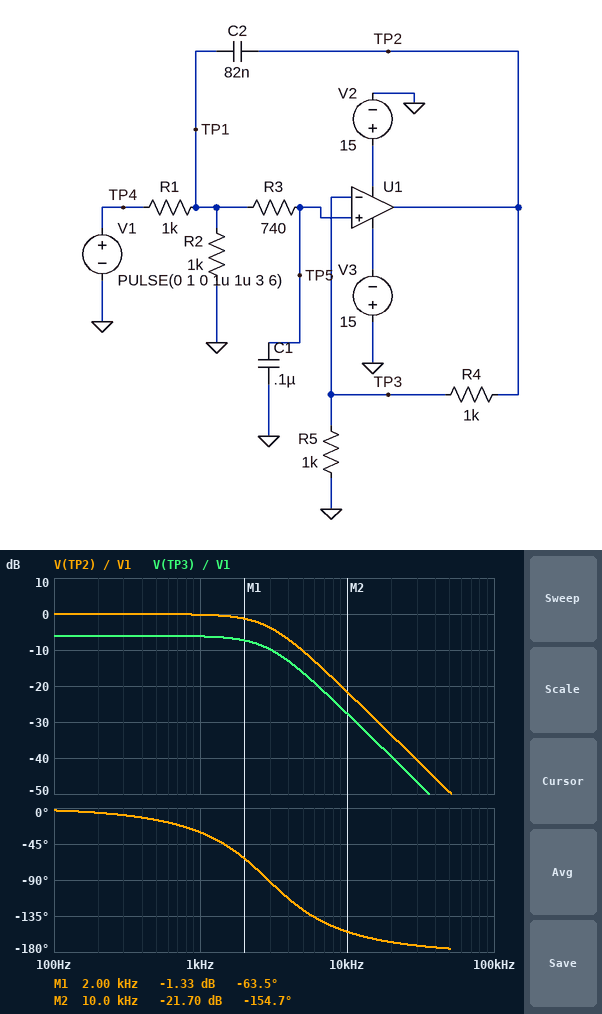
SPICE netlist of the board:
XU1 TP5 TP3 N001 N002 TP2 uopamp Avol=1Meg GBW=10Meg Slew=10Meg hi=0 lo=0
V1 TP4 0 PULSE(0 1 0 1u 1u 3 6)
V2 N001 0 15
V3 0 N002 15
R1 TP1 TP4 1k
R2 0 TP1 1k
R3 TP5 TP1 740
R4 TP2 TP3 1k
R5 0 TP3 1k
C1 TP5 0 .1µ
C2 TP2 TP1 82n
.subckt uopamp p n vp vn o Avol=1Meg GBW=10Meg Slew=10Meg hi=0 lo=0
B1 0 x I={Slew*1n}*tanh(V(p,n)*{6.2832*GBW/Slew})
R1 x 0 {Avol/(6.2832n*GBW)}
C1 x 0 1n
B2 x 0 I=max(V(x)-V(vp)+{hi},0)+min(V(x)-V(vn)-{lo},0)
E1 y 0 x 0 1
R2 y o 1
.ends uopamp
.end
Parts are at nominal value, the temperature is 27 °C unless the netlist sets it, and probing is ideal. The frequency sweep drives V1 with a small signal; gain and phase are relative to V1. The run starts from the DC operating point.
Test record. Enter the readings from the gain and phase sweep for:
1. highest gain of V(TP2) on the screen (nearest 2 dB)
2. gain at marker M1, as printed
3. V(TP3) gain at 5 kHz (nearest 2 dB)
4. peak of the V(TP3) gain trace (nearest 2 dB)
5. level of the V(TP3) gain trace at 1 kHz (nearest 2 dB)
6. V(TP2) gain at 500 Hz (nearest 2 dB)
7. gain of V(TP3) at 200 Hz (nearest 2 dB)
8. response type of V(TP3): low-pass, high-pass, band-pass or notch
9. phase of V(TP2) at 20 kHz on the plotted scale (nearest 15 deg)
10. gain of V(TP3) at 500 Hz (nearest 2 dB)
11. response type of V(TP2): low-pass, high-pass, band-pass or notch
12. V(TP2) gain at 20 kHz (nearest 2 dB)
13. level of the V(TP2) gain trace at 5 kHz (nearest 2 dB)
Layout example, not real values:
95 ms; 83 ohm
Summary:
0 dB; -1.33 dB; -16 dB; -6 dB; -6 dB; 0 dB; -6 dB; low-pass; -165 deg; -6 dB; low-pass; -34 dB; -10 dB
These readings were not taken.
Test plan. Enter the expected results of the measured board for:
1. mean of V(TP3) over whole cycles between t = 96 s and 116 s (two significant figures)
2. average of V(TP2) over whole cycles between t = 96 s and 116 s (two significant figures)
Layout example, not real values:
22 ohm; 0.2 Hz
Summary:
250 mV; 500 mV
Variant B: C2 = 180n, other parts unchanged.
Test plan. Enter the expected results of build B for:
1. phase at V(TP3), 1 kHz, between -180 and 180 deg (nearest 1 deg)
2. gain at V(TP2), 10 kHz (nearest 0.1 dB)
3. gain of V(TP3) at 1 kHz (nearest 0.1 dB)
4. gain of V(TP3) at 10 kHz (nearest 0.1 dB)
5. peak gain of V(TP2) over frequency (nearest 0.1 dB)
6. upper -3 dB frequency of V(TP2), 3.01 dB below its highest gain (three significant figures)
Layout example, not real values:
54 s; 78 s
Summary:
-16 deg; -28.1 dB; -3.7 dB; -34.1 dB; 7.8 dB; 2.24 kHz
